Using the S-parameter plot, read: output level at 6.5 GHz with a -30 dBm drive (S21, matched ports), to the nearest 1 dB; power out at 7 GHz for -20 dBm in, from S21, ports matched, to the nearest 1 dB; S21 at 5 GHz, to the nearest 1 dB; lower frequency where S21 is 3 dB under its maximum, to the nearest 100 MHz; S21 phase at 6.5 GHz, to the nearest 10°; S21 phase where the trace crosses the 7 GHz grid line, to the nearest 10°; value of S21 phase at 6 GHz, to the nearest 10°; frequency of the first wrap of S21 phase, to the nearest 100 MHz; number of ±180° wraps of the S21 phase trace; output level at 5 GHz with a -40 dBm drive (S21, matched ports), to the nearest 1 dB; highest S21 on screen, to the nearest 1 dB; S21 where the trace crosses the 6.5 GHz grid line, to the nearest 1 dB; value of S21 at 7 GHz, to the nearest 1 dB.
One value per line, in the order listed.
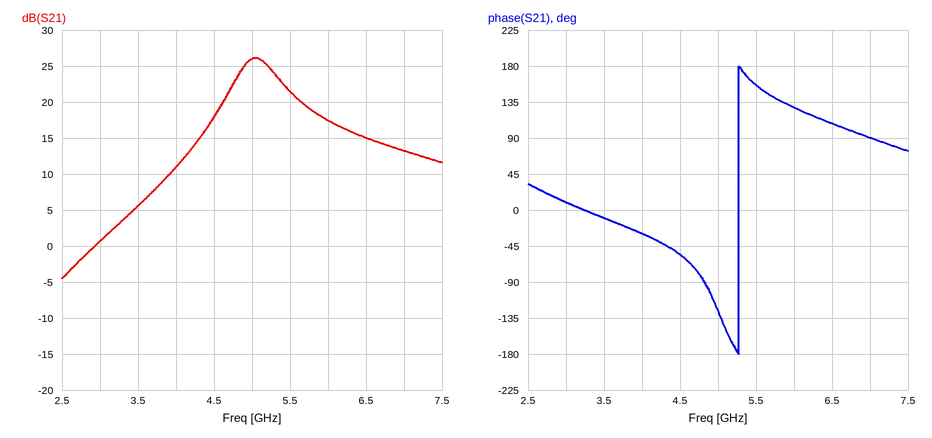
-15 dBm
-7 dBm
26 dB
4.8 GHz
110°
90°
130°
5.3 GHz
1
-14 dBm
26 dB
15 dB
13 dB
